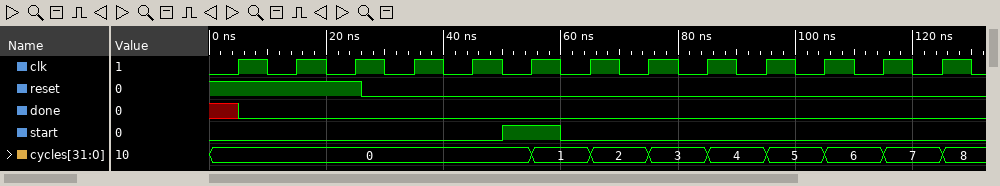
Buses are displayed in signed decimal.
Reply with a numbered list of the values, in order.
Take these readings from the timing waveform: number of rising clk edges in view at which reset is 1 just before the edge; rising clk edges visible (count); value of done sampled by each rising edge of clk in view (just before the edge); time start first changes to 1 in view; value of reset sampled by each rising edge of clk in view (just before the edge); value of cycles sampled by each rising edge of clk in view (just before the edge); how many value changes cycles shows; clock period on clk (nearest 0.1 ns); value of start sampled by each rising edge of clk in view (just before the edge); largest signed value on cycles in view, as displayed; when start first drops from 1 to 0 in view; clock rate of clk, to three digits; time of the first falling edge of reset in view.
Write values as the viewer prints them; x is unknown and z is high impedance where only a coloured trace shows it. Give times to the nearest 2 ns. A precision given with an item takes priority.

1. 3
2. 13
3. x 0 0 0 0 0 0 0 0 0 0 0 0
4. 50 ns
5. 1 1 1 0 0 0 0 0 0 0 0 0 0
6. 0, 0, 0, 0, 0, 0, 1, 2, 3, 4, 5, 6, 7
7. 8
8. 10 ns
9. 0 0 0 0 0 1 0 0 0 0 0 0 0
10. 8
11. 60 ns
12. 100 MHz
13. 26 ns
